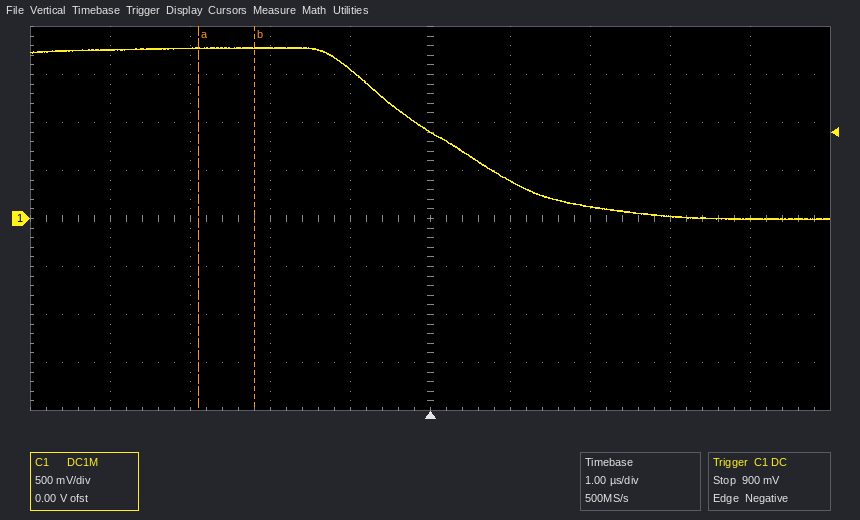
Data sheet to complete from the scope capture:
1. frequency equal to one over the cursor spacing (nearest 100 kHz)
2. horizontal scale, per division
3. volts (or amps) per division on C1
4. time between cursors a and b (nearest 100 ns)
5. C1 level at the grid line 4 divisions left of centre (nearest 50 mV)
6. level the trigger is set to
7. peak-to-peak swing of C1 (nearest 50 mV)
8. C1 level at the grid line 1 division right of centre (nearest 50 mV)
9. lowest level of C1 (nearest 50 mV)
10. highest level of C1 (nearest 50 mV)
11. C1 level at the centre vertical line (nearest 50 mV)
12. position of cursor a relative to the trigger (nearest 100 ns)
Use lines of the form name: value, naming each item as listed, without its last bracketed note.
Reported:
frequency equal to one over the cursor spacing: 1.4 MHz
horizontal scale, per division: 1 µs
volts (or amps) per division on C1: 500 mV
time between cursors a and b: 700 ns
C1 level at the grid line 4 divisions left of centre: 1.75 V
level the trigger is set to: 900 mV
peak-to-peak swing of C1: 1.80 V
C1 level at the grid line 1 division right of centre: 400 mV
lowest level of C1: 0 mV
highest level of C1: 1.80 V
C1 level at the centre vertical line: 900 mV
position of cursor a relative to the trigger: -2.9 µs
